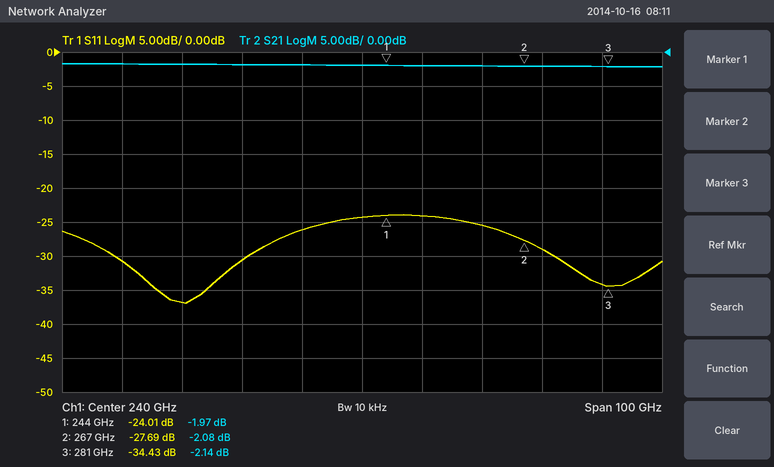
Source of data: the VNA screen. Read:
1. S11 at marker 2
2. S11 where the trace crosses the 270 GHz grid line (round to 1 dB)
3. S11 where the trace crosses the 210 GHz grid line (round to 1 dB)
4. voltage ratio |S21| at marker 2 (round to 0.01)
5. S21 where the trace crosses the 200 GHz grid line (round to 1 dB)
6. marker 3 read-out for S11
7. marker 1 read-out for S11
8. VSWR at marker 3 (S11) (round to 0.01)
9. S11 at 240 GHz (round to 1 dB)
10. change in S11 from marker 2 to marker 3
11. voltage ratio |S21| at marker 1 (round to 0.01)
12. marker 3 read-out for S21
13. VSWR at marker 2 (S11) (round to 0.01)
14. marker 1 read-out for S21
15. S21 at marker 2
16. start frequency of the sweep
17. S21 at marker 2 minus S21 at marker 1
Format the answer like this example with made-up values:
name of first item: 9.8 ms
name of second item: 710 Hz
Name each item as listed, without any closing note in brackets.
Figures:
S11 at marker 2: -27.69 dB
S11 where the trace crosses the 270 GHz grid line: -29 dB
S11 where the trace crosses the 210 GHz grid line: -37 dB
voltage ratio |S21| at marker 2: 0.79
S21 where the trace crosses the 200 GHz grid line: -2 dB
marker 3 read-out for S11: -34.43 dB
marker 1 read-out for S11: -24.01 dB
VSWR at marker 3 (S11): 1.04
S11 at 240 GHz: -24 dB
change in S11 from marker 2 to marker 3: -6.74 dB
voltage ratio |S21| at marker 1: 0.80
marker 3 read-out for S21: -2.14 dB
VSWR at marker 2 (S11): 1.09
marker 1 read-out for S21: -1.97 dB
S21 at marker 2: -2.08 dB
start frequency of the sweep: 190 GHz
S21 at marker 2 minus S21 at marker 1: -0.11 dB
